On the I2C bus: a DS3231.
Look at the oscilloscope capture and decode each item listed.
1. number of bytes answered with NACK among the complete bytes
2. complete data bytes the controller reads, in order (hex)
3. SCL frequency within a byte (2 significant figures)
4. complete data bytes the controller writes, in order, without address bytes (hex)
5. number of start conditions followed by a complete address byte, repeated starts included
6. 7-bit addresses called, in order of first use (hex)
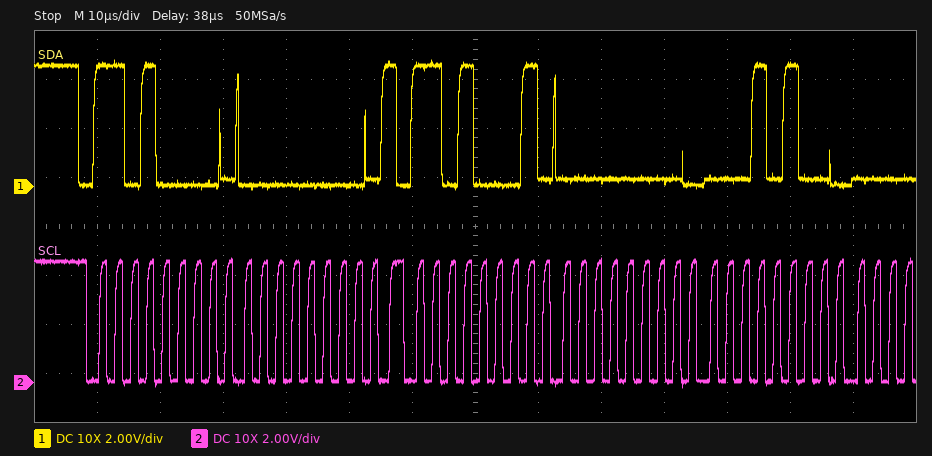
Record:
0
00 14
400 kHz
00
2
0x68
